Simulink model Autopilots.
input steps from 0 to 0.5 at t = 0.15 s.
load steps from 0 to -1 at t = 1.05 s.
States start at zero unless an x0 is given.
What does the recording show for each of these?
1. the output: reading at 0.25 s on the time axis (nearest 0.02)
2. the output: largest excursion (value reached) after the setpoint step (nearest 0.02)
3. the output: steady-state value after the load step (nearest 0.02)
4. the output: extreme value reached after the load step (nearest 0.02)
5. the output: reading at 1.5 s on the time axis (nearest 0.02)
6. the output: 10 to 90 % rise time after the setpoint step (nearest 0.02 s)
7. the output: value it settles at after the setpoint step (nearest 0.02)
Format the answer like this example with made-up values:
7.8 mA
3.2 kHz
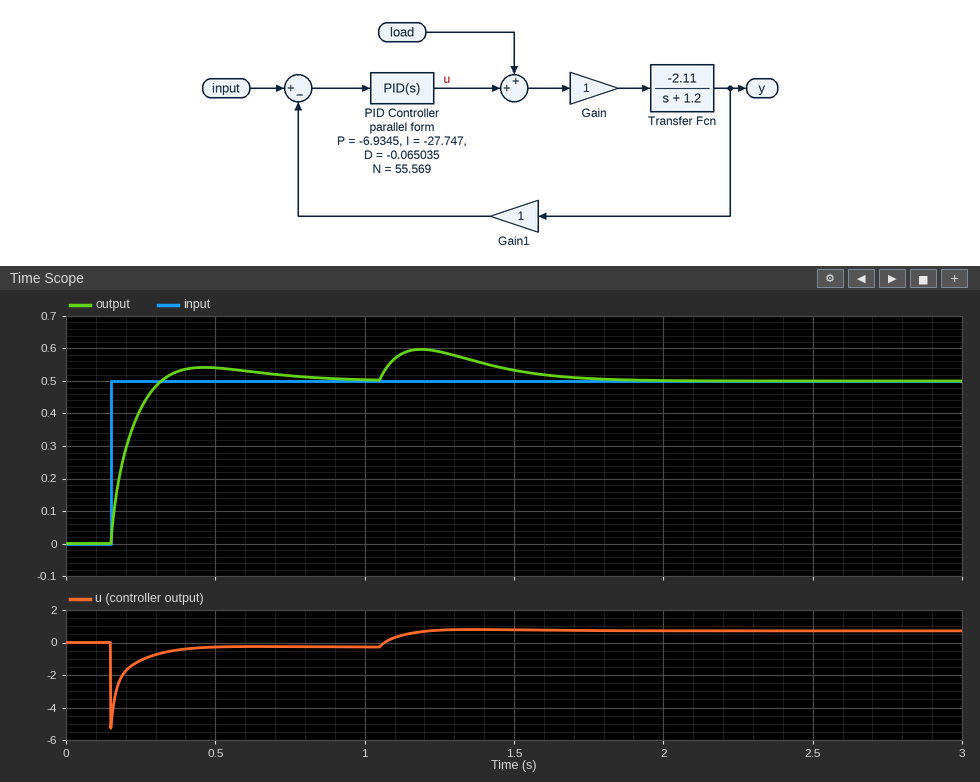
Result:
0.42
0.54
0.50
0.60
0.54
0.12 s
0.50
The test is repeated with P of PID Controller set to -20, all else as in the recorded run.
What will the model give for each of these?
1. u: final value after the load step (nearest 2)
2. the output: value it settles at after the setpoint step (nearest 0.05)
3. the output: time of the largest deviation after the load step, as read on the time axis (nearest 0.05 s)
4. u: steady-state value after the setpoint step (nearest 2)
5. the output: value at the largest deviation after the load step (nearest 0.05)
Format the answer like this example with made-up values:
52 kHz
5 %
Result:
0
0.50
1.15 s
0
0.55
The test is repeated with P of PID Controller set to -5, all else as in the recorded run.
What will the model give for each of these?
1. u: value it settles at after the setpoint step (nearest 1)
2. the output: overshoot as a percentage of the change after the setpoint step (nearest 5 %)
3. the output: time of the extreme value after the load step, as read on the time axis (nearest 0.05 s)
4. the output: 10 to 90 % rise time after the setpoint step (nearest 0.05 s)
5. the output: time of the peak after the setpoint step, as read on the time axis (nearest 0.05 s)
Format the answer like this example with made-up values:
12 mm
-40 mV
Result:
0
15 %
1.20 s
0.15 s
0.50 s
